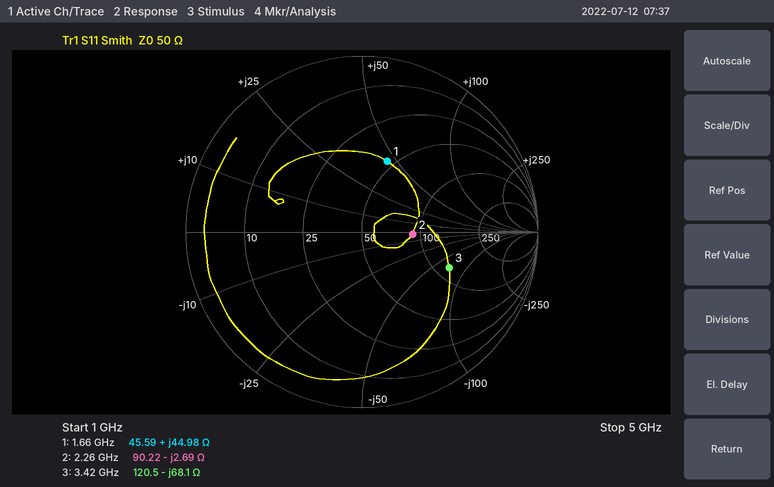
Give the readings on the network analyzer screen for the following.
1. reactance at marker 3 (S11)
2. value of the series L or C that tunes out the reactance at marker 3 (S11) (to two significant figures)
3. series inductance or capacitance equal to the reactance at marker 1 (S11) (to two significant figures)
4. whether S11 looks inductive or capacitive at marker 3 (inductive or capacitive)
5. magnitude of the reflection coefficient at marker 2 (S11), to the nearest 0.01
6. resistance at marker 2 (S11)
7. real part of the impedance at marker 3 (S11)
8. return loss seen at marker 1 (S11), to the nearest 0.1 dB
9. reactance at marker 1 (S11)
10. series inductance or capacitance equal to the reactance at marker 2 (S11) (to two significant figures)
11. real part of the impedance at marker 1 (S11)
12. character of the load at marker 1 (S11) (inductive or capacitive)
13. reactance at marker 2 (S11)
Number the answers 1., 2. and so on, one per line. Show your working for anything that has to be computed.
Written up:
1. -68.1 Ω
2. L = 68.1 Ω/(2π × 3.42 GHz) ≈ 3.2 nH
3. L = 44.98 Ω/(2π × 1.66 GHz) ≈ 4.3 nH
4. capacitive
5. 0.29
6. 90.22 Ω
7. 120.5 Ω
8. 7.4 dB
9. +44.98 Ω
10. C = 1/(2π × 2.26 GHz × 2.69 Ω) ≈ 26 pF
11. 45.59 Ω
12. inductive
13. -2.69 Ω
